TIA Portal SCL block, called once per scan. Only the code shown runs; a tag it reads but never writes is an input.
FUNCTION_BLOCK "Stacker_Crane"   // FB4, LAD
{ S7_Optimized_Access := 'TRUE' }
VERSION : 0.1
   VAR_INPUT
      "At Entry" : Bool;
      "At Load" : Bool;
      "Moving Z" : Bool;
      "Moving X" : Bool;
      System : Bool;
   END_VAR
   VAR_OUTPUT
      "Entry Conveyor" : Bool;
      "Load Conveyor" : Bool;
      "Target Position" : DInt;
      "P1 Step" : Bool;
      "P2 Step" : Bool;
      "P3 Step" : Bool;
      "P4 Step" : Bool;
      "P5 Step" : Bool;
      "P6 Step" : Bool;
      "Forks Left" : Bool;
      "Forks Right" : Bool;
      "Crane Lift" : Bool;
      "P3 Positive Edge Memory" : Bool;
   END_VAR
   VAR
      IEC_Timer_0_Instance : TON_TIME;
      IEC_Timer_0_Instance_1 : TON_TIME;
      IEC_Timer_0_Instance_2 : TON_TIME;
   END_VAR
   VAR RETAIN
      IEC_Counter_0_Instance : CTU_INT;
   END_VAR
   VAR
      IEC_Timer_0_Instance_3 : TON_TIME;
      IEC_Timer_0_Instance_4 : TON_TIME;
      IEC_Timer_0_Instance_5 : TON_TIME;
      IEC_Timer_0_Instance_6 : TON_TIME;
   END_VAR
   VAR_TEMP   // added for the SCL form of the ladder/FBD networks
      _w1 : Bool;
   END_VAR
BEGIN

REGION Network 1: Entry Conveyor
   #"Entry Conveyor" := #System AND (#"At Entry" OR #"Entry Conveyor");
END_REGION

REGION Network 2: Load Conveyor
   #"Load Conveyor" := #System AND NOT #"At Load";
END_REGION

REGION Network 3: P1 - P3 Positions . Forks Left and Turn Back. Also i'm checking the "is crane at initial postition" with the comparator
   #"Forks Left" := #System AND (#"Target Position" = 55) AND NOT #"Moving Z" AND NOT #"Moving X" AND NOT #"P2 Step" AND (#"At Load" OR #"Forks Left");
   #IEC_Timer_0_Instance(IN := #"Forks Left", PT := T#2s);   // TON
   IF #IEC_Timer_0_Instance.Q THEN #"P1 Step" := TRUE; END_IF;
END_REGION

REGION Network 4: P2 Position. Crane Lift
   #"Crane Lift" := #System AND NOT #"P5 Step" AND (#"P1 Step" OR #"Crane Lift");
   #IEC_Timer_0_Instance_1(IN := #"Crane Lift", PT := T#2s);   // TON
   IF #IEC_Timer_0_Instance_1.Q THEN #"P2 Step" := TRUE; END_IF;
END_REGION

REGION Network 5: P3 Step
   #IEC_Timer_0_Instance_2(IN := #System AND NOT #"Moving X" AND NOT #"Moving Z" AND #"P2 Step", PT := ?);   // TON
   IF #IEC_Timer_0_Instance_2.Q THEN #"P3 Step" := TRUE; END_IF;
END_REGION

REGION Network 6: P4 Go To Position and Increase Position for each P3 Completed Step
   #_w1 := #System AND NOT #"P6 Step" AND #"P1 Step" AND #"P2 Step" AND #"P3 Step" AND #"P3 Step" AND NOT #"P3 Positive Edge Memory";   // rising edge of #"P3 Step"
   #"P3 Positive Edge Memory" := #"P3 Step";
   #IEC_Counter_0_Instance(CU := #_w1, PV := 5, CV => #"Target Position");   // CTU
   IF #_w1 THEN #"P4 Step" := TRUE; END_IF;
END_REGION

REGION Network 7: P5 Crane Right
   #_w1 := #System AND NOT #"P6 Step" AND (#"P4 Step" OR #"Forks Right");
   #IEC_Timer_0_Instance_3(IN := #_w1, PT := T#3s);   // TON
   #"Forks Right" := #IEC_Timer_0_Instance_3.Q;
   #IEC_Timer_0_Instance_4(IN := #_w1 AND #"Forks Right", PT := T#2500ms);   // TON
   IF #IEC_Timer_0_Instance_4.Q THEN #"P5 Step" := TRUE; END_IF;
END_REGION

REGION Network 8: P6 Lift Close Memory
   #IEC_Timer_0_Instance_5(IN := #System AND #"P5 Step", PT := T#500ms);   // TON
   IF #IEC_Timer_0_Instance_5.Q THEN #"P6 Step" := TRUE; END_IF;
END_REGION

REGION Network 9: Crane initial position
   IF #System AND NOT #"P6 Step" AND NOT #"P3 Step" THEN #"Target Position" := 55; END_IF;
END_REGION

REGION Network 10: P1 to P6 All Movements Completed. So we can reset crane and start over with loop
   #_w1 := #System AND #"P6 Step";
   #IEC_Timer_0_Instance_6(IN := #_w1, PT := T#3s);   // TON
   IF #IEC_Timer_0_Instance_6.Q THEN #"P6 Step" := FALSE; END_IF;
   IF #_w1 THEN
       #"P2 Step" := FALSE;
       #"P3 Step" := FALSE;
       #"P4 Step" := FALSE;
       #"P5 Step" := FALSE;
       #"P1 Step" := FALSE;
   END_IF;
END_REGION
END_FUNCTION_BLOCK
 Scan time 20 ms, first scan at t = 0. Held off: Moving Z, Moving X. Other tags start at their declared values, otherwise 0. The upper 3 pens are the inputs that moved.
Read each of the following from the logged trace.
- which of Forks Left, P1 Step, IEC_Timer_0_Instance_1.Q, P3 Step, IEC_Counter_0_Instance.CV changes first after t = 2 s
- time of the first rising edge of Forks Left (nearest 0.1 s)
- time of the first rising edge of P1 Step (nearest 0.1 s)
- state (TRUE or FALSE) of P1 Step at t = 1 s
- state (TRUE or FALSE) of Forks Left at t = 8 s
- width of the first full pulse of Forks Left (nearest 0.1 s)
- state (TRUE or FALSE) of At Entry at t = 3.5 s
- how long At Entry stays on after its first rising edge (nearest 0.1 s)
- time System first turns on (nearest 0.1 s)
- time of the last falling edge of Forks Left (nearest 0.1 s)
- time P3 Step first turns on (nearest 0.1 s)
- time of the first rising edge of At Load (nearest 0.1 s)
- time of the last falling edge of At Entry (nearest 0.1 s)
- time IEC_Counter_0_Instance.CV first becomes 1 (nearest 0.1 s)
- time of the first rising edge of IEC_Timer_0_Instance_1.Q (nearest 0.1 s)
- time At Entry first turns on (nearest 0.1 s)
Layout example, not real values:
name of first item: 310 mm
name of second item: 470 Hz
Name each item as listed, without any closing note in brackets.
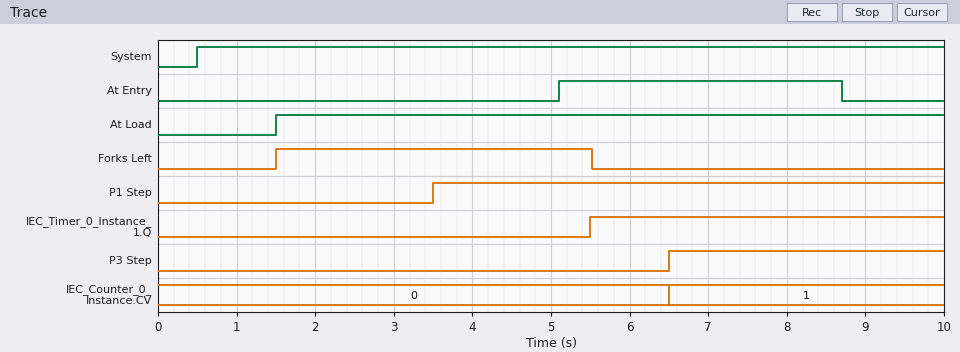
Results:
which of Forks Left, P1 Step, IEC_Timer_0_Instance_1.Q, P3 Step, IEC_Counter_0_Instance.CV changes first after t = 2 s: P1 Step
time of the first rising edge of Forks Left: 1.5 s
time of the first rising edge of P1 Step: 3.5 s
state (TRUE or FALSE) of P1 Step at t = 1 s: FALSE
state (TRUE or FALSE) of Forks Left at t = 8 s: FALSE
width of the first full pulse of Forks Left: 4.0 s
state (TRUE or FALSE) of At Entry at t = 3.5 s: FALSE
how long At Entry stays on after its first rising edge: 3.6 s
time System first turns on: 0.5 s
time of the last falling edge of Forks Left: 5.5 s
time P3 Step first turns on: 6.5 s
time of the first rising edge of At Load: 1.5 s
time of the last falling edge of At Entry: 8.7 s
time IEC_Counter_0_Instance.CV first becomes 1: 6.5 s
time of the first rising edge of IEC_Timer_0_Instance_1.Q: 5.5 s
time At Entry first turns on: 5.1 s
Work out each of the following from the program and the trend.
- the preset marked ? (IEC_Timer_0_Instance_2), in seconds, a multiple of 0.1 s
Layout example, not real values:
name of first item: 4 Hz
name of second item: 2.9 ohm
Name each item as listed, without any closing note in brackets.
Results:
the preset marked ? (IEC_Timer_0_Instance_2), in seconds, a multiple of 0.1 s: 1.0 s
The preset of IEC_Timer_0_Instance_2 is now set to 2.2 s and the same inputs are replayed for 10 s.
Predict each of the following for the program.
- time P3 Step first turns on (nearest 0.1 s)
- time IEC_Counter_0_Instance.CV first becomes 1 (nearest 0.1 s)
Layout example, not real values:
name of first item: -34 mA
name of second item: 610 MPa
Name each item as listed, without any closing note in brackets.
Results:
time P3 Step first turns on: 7.7 s
time IEC_Counter_0_Instance.CV first becomes 1: 7.7 s
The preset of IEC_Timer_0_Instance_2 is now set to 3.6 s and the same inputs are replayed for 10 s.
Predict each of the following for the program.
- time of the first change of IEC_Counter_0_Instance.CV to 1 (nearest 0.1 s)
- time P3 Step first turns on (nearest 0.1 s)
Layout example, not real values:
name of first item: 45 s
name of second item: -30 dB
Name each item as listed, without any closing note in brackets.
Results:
time of the first change of IEC_Counter_0_Instance.CV to 1: 9.1 s
time P3 Step first turns on: 9.1 s
